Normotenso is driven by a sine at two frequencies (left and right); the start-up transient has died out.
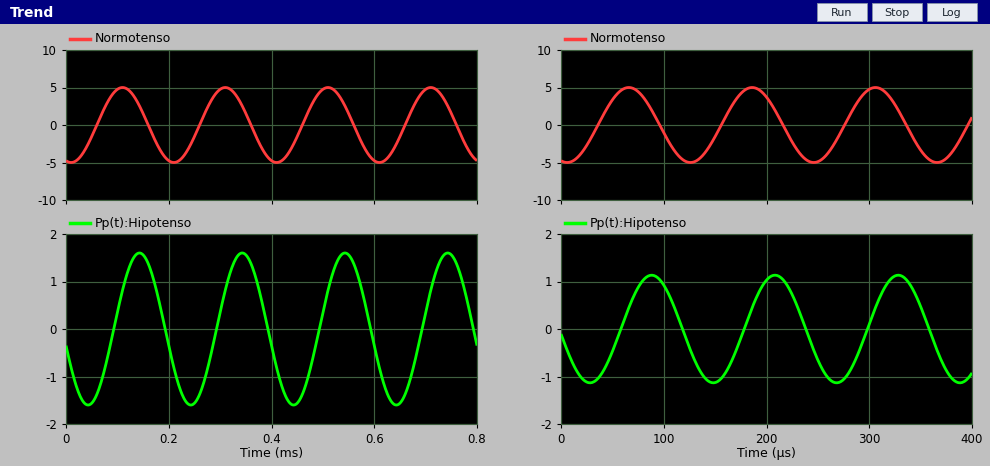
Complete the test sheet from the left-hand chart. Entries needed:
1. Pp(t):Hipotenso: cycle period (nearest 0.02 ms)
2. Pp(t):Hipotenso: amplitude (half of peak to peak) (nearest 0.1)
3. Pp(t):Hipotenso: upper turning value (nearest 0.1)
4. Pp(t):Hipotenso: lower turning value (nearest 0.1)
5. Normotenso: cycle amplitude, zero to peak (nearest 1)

0.20 ms
1.6
1.6
-1.6
5
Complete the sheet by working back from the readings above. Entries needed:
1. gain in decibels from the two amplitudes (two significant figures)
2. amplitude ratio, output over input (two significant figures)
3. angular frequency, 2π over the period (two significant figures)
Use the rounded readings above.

-9.9 dB
0.32
31 rad/ms
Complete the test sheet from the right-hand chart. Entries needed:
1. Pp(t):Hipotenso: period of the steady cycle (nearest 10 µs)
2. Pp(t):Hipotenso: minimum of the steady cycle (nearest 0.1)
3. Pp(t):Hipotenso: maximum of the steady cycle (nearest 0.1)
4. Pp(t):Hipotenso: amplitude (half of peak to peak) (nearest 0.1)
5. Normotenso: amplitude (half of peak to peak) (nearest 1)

120 µs
-1.1
1.1
1.1
5
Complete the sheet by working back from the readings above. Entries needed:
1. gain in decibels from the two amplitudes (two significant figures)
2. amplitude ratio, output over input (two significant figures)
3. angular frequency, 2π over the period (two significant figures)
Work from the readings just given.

-13 dB
0.22
0.052 rad/µs
